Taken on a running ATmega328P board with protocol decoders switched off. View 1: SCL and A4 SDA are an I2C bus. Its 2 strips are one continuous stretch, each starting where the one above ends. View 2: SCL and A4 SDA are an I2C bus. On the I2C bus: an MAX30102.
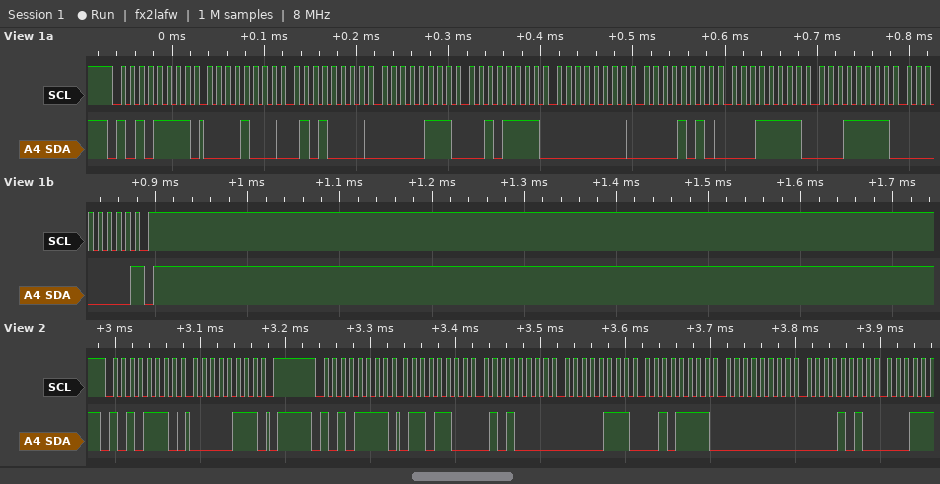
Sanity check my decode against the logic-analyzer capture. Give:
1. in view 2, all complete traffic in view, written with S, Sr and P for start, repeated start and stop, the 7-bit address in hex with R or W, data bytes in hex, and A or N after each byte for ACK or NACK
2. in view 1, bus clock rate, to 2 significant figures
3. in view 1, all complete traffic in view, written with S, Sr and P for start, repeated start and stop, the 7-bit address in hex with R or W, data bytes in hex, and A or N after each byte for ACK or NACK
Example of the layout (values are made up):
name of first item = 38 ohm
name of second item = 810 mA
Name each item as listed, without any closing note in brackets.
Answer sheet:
in view 2, all complete traffic in view, written with S, Sr and P for start, repeated start and stop, the 7-bit address in hex with R or W, data bytes in hex, and A or N after each byte for ACK or NACK = S 57W A 07 A P S 57R A 6C A 50 A 07 A 2F A 00 A 0A A
in view 1, bus clock rate, to 2 significant figures = 100 kHz
in view 1, all complete traffic in view, written with S, Sr and P for start, repeated start and stop, the 7-bit address in hex with R or W, data bytes in hex, and A or N after each byte for ACK or NACK = S 57R A 08 A 50 A 07 A 2F A 00 A 0A A 1F A 1F A 00 N P
